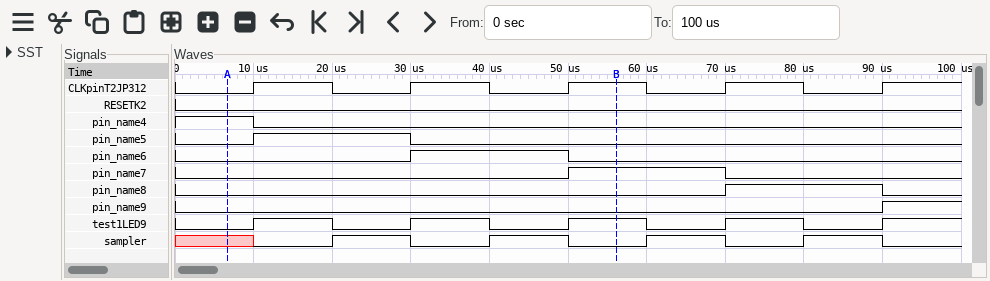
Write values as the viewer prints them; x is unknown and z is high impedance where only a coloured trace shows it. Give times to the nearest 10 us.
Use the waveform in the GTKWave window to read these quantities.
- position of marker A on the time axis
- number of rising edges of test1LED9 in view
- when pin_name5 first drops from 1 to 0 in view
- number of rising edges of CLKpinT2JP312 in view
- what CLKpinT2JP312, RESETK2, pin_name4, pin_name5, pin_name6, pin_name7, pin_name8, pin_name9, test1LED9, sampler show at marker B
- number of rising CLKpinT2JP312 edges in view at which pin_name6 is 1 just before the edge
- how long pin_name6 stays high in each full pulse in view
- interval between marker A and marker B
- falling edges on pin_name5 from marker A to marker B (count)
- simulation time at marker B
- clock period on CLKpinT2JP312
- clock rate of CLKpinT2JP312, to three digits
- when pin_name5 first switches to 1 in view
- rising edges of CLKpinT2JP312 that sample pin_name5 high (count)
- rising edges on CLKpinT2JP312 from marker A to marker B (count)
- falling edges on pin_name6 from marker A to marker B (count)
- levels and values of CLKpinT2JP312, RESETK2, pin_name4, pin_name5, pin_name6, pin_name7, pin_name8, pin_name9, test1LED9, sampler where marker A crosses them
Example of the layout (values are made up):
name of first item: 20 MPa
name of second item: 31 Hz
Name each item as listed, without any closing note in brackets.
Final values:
position of marker A on the time axis: 10 us
number of rising edges of test1LED9 in view: 5
when pin_name5 first drops from 1 to 0 in view: 30 us
number of rising edges of CLKpinT2JP312 in view: 5
what CLKpinT2JP312, RESETK2, pin_name4, pin_name5, pin_name6, pin_name7, pin_name8, pin_name9, test1LED9, sampler show at marker B: CLKpinT2JP312=1, RESETK2=0, pin_name4=0, pin_name5=0, pin_name6=0, pin_name7=1, pin_name8=0, pin_name9=0, test1LED9=1, sampler=0
number of rising CLKpinT2JP312 edges in view at which pin_name6 is 1 just before the edge: 1
how long pin_name6 stays high in each full pulse in view: 20 us
interval between marker A and marker B: 50 us
falling edges on pin_name5 from marker A to marker B: 1
simulation time at marker B: 60 us
clock period on CLKpinT2JP312: 20 us
clock rate of CLKpinT2JP312, to three digits: 50.0 kHz
when pin_name5 first switches to 1 in view: 10 us
rising edges of CLKpinT2JP312 that sample pin_name5 high: 1
rising edges on CLKpinT2JP312 from marker A to marker B: 3
falling edges on pin_name6 from marker A to marker B: 1
levels and values of CLKpinT2JP312, RESETK2, pin_name4, pin_name5, pin_name6, pin_name7, pin_name8, pin_name9, test1LED9, sampler where marker A crosses them: CLKpinT2JP312=0, RESETK2=0, pin_name4=1, pin_name5=0, pin_name6=0, pin_name7=0, pin_name8=0, pin_name9=0, test1LED9=0, sampler=x
